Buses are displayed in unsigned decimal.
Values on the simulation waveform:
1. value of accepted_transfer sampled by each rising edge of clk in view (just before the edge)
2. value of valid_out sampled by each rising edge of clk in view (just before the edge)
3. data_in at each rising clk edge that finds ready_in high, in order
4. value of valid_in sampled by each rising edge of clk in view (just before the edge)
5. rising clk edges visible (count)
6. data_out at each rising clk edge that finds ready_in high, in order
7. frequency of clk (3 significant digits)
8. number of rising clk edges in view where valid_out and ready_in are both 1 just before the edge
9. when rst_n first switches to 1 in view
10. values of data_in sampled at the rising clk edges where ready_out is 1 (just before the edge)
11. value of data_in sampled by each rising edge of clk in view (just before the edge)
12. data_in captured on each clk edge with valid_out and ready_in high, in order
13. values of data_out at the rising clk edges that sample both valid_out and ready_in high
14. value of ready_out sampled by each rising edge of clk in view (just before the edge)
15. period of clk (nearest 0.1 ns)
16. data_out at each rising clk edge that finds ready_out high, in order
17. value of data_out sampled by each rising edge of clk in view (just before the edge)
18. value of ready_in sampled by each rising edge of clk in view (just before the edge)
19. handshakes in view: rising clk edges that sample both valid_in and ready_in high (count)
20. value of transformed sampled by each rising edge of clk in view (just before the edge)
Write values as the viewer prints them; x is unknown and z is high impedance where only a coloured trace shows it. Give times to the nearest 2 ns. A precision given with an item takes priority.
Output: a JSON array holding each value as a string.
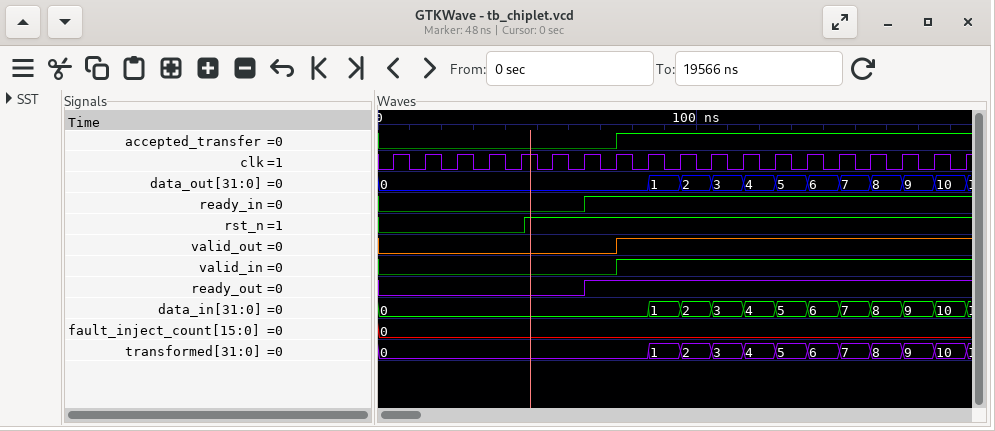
["0 0 0 0 0 0 0 0 1 1 1 1 1 1 1 1 1 1 1", "0 0 0 0 0 0 0 0 1 1 1 1 1 1 1 1 1 1 1", "0, 0, 1, 2, 3, 4, 5, 6, 7, 8, 9, 10", "0 0 0 0 0 0 0 0 1 1 1 1 1 1 1 1 1 1 1", "19", "0, 0, 1, 2, 3, 4, 5, 6, 7, 8, 9, 10", "100 MHz", "11", "46 ns", "0, 0, 1, 2, 3, 4, 5, 6, 7, 8, 9, 10", "0, 0, 0, 0, 0, 0, 0, 0, 0, 1, 2, 3, 4, 5, 6, 7, 8, 9, 10", "0, 1, 2, 3, 4, 5, 6, 7, 8, 9, 10", "0, 1, 2, 3, 4, 5, 6, 7, 8, 9, 10", "0 0 0 0 0 0 0 1 1 1 1 1 1 1 1 1 1 1 1", "10 ns", "0, 0, 1, 2, 3, 4, 5, 6, 7, 8, 9, 10", "0, 0, 0, 0, 0, 0, 0, 0, 0, 1, 2, 3, 4, 5, 6, 7, 8, 9, 10", "0 0 0 0 0 0 0 1 1 1 1 1 1 1 1 1 1 1 1", "11", "0, 0, 0, 0, 0, 0, 0, 0, 0, 1, 2, 3, 4, 5, 6, 7, 8, 9, 10"]
